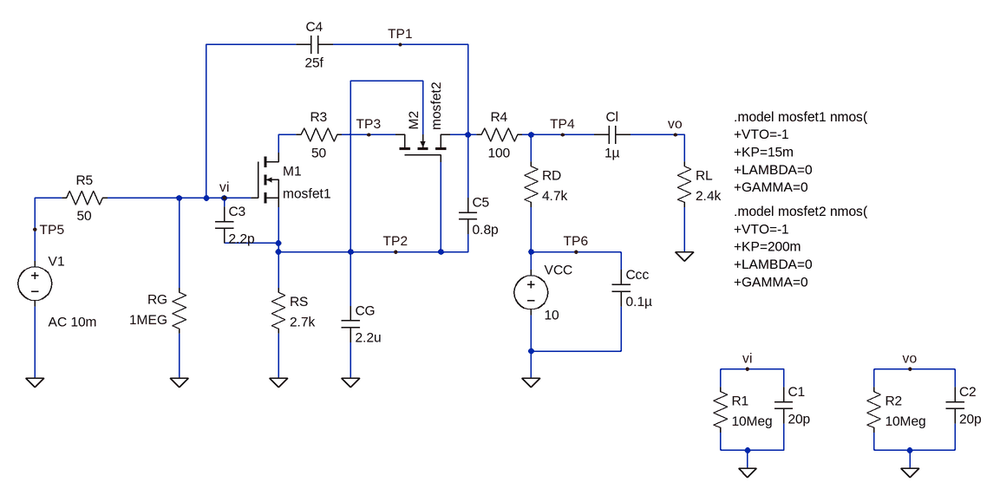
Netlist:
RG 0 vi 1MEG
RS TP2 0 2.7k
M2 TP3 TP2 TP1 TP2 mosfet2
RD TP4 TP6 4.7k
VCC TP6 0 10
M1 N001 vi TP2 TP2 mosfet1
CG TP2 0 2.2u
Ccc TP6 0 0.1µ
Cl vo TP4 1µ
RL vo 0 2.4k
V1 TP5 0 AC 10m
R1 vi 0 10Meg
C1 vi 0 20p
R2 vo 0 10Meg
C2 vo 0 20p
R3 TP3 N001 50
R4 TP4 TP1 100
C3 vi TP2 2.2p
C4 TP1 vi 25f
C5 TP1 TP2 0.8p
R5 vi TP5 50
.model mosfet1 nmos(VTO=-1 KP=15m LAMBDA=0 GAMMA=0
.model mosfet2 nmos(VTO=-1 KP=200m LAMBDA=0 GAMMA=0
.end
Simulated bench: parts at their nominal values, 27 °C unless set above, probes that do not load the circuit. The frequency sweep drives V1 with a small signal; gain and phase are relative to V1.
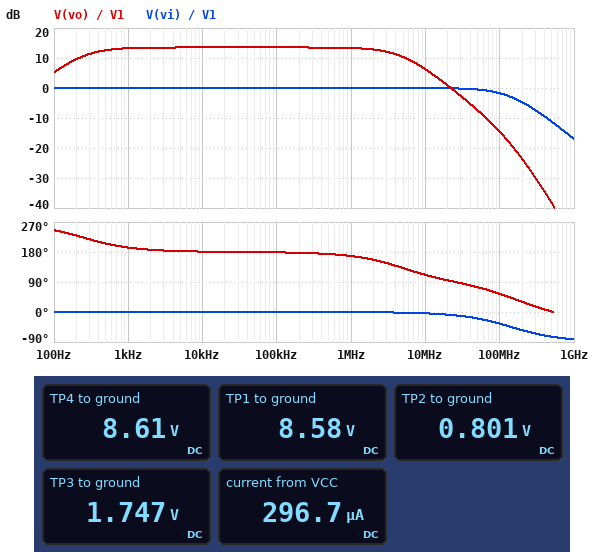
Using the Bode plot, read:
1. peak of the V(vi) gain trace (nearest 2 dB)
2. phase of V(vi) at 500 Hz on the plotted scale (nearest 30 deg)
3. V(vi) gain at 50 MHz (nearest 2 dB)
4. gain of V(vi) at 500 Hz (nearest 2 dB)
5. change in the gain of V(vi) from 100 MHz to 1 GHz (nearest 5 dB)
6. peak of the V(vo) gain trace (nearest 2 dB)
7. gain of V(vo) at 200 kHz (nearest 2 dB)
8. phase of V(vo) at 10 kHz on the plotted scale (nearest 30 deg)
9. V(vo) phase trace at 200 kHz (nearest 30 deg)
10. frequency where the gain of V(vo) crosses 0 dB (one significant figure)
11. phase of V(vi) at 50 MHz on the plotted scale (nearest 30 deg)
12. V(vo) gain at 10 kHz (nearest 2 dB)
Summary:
0 dB
0 deg
0 dB
0 dB
-15 dB
14 dB
14 dB
180 deg
180 deg
20 MHz
-30 deg
14 dB
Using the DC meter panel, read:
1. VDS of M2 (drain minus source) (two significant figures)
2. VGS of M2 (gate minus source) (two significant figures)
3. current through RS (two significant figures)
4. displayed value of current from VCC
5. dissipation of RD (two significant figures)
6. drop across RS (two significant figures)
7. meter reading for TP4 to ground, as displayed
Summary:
-6.8 V
-7.8 V
300 µA
296.7 µA
410 µW
800 mV
8.61 V
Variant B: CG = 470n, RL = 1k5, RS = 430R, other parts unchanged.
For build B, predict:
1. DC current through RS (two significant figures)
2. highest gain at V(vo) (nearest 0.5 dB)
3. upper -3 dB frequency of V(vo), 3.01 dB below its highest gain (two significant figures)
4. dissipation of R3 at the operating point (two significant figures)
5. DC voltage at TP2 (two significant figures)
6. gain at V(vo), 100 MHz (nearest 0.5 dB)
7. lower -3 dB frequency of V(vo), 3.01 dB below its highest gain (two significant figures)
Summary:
1.3 mA
17.0 dB
6.7 MHz
90 µW
580 mV
-8.0 dB
2.7 kHz
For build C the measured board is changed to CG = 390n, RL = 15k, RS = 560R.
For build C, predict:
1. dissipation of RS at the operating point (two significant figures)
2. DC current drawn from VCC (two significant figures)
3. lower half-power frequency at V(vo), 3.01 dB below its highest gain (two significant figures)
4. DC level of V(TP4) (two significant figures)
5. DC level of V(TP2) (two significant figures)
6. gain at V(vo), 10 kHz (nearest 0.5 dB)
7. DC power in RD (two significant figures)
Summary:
680 µW
1.1 mA
2.9 kHz
4.8 V
620 mV
26.0 dB
5.7 mW
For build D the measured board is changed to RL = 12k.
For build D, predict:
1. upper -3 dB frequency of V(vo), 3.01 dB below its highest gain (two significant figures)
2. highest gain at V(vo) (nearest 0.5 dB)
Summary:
2.3 MHz
20.0 dB
